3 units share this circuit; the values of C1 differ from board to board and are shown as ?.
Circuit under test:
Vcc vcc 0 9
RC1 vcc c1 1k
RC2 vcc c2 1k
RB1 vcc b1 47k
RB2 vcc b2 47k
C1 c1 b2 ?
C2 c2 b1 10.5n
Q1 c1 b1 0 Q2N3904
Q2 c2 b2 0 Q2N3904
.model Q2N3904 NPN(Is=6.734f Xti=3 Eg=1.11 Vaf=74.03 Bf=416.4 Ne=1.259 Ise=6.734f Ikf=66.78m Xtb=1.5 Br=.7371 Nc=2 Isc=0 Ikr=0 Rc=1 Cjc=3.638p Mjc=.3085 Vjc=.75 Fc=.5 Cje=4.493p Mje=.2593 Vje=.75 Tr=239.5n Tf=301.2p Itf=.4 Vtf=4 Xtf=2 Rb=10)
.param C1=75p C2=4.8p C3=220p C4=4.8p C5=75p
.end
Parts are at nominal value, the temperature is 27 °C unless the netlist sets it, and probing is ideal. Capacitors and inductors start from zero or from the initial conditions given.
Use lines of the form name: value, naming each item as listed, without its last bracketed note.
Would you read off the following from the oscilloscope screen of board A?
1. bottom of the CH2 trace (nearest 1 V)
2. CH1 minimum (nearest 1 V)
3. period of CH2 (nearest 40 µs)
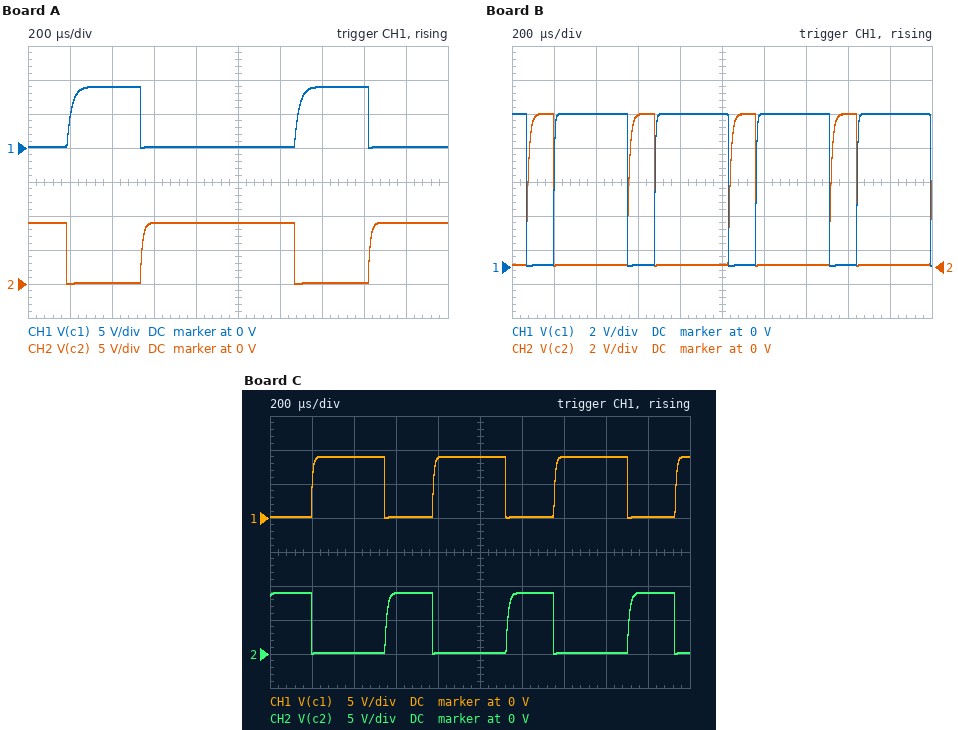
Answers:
bottom of the CH2 trace: 0 V
CH1 minimum: 0 V
period of CH2: 1.08 ms
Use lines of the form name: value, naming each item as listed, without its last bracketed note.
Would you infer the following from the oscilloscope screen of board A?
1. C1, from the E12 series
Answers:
C1, from the E12 series: 22 nF
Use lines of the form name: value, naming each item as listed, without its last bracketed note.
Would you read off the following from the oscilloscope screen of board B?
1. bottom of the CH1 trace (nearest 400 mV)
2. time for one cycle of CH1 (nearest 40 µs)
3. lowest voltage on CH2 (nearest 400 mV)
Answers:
bottom of the CH1 trace: 0 V
time for one cycle of CH1: 480 µs
lowest voltage on CH2: 0 V
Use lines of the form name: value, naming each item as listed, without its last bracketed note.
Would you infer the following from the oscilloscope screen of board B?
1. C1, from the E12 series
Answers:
C1, from the E12 series: 3.9 nF
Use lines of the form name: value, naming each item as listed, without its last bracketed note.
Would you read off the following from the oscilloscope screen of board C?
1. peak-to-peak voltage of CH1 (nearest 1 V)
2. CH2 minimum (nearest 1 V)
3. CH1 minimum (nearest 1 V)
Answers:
peak-to-peak voltage of CH1: 9 V
CH2 minimum: 0 V
CH1 minimum: 0 V
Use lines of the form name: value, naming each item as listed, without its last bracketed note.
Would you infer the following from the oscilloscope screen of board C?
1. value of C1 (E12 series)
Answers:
value of C1: 6.8 nF
